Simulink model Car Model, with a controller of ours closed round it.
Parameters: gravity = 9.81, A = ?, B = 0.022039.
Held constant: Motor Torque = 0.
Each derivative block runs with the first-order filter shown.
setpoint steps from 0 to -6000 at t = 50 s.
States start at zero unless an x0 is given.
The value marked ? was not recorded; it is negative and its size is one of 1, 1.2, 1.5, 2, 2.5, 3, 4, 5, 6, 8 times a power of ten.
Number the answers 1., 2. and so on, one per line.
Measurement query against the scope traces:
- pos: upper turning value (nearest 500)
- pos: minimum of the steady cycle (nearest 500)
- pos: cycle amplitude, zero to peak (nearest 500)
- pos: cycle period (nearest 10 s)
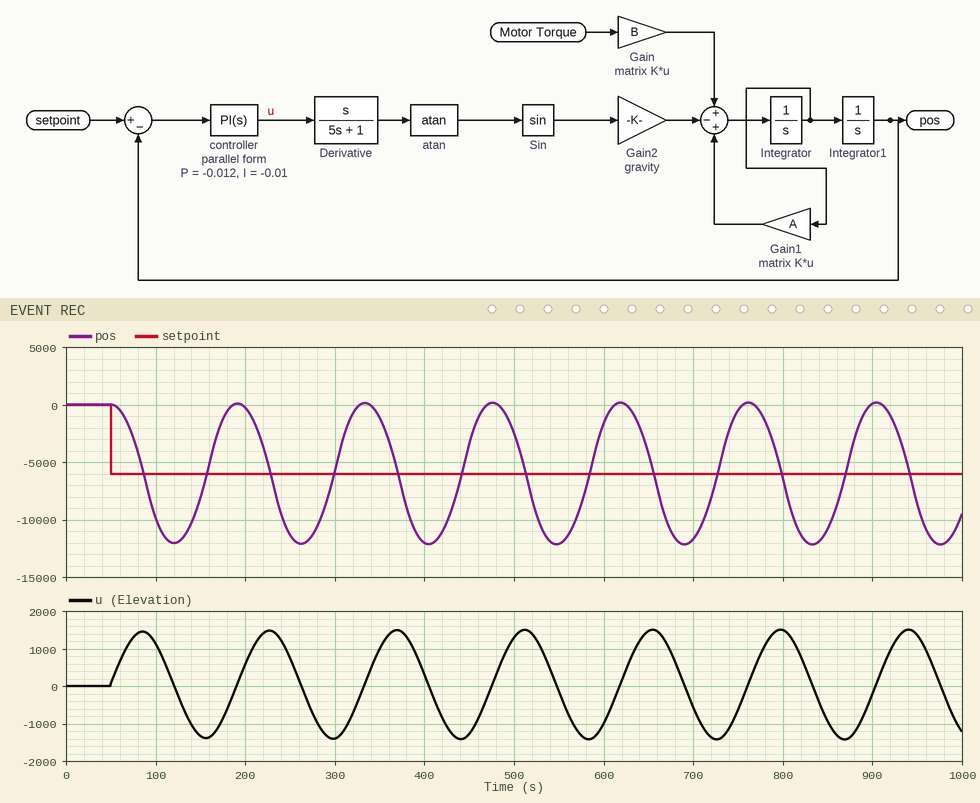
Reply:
1. 0
2. -12000
3. 6000
4. 140 s
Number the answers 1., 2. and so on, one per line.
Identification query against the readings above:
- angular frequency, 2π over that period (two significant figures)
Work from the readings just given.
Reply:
1. 0.045 rad/s
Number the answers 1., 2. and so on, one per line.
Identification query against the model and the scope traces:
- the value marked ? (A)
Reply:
1. -0.008
